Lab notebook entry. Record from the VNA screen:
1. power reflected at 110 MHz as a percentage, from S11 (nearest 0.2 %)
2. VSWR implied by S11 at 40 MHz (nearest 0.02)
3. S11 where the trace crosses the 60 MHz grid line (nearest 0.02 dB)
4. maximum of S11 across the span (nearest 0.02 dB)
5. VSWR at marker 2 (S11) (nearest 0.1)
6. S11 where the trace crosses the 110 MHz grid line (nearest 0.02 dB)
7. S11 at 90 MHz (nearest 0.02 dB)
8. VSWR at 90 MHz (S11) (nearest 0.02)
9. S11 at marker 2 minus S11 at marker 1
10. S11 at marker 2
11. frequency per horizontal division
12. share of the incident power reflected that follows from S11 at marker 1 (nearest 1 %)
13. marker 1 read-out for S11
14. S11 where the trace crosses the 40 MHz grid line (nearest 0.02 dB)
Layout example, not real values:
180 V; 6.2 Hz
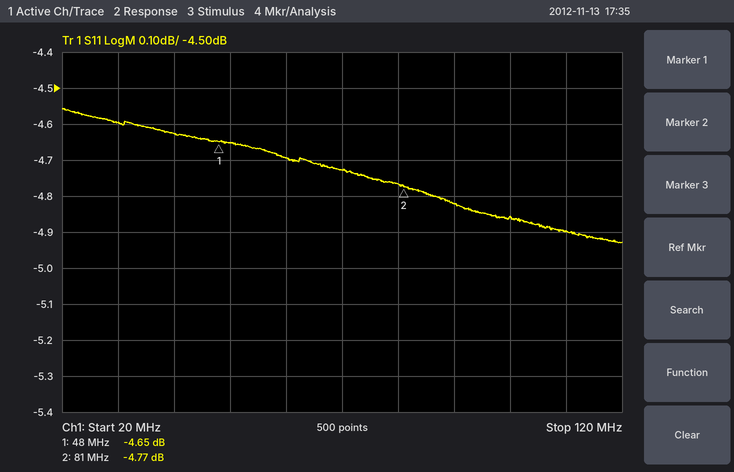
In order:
32.4 %; 3.84; -4.70 dB; -4.56 dB; 3.7; -4.90 dB; -4.82 dB; 3.70; -0.12 dB; -4.77 dB; 10 MHz; 34 %; -4.65 dB; -4.62 dB
